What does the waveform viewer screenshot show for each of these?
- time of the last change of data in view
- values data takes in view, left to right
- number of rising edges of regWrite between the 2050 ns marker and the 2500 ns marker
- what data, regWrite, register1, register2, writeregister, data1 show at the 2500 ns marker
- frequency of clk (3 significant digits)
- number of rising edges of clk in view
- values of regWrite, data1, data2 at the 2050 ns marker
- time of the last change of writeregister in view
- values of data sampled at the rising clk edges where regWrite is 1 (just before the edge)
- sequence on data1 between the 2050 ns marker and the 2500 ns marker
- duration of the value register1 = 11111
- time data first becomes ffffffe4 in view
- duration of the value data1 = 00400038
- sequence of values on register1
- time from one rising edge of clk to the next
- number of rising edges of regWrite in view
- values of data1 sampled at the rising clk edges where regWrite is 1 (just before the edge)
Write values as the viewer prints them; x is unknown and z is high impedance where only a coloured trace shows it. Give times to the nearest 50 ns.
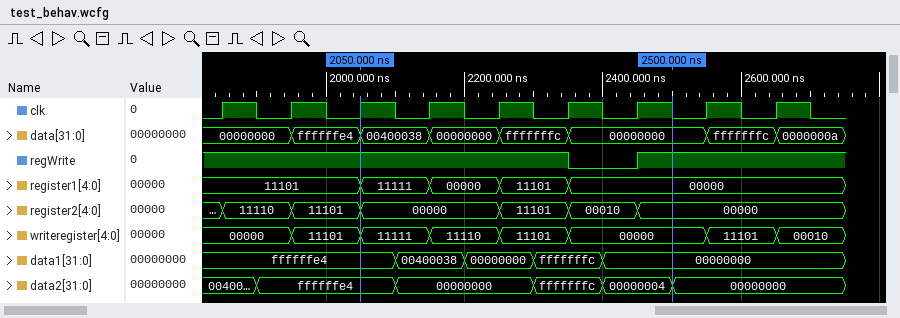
2650 ns
00000000, ffffffe4, 00400038, 00000000, fffffffc, 00000000, fffffffc, 0000000a
1
data=00000000, regWrite=1, register1=00000, register2=00000, writeregister=00000, data1=00000000
10.0 MHz
9
regWrite=1, data1=ffffffe4, data2=ffffffe4
2650 ns
00000000, 00000000, ffffffe4, 00400038, 00000000, fffffffc, 00000000, fffffffc
ffffffe4, 00400038, 00000000, fffffffc, 00000000
100 ns
1950 ns
100 ns
11101, 11111, 00000, 11101, 00000
100 ns
1
ffffffe4, ffffffe4, ffffffe4, 00400038, 00000000, fffffffc, 00000000, 00000000
